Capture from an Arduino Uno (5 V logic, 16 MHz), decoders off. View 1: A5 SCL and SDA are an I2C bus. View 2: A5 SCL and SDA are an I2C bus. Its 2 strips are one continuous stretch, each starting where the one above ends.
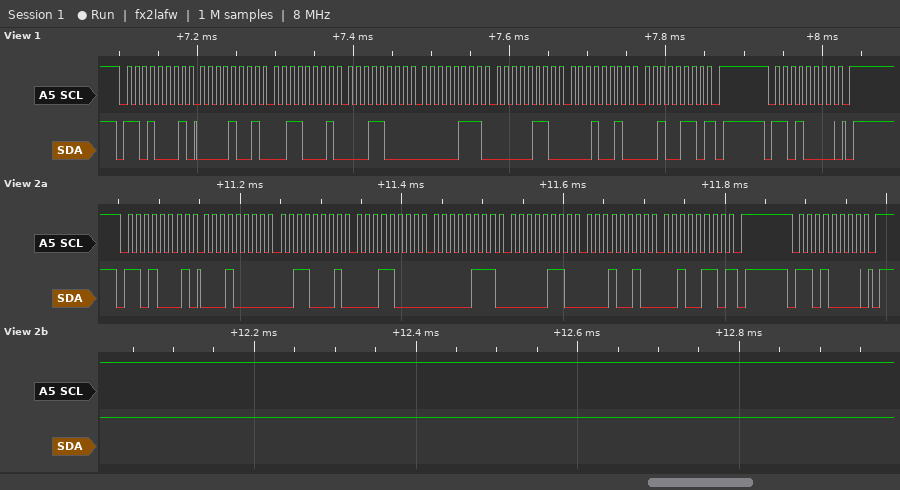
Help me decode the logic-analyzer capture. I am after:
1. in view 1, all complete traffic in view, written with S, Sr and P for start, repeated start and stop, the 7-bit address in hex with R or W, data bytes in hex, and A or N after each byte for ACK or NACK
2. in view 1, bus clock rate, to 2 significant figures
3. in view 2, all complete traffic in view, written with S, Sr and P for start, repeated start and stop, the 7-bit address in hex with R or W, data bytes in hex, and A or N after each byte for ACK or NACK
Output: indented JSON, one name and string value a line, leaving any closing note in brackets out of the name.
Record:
{
  "in view 1, all complete traffic in view, written with S, Sr and P for start, repeated start and stop, the 7-bit address in hex with R or W, data bytes in hex, and A or N after each byte for ACK or NACK": "S 68R A 09 A 31 A 18 A 07 A 06 A 12 A 26 N P S 68W A P",
  "in view 1, bus clock rate, to 2 significant figures": "100 kHz",
  "in view 2, all complete traffic in view, written with S, Sr and P for start, repeated start and stop, the 7-bit address in hex with R or W, data bytes in hex, and A or N after each byte for ACK or NACK": "S 68R A 10 A 31 A 18 A 07 A 06 A 12 A 26 N P S 68W A P"
}
